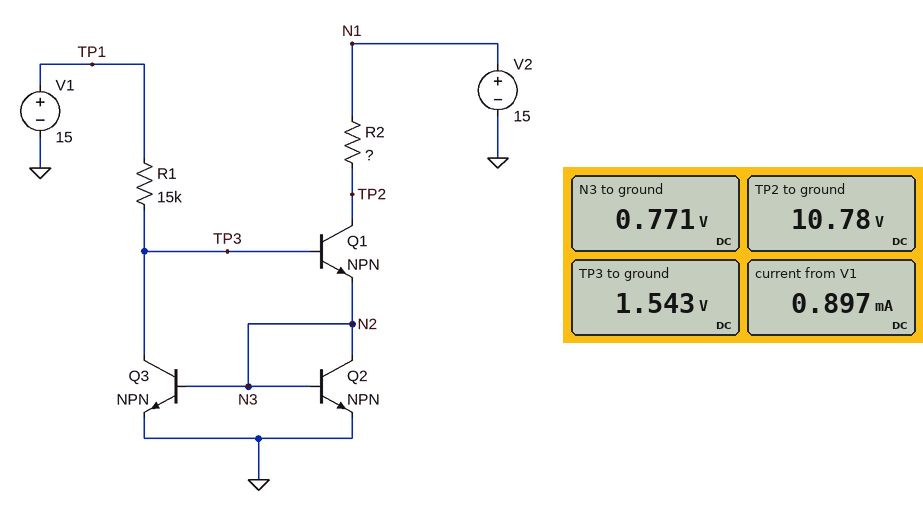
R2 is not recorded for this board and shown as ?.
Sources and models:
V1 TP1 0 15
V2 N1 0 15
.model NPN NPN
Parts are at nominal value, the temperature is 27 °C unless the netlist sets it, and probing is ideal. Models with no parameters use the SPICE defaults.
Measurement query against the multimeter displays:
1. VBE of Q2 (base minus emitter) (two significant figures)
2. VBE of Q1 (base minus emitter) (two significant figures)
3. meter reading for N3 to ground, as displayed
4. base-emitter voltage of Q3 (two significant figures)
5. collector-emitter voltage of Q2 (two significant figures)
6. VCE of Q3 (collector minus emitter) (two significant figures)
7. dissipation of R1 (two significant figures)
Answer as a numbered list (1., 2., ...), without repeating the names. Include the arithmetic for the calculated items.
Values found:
1. 771 mV = 770 mV
2. 1.543 V - 771 mV = 770 mV
3. 0.771 V
4. 771 mV = 770 mV
5. 771 mV = 770 mV
6. 1.543 V = 1.5 V
7. (15 V - 1.543 V)^2 / 15 kΩ = 12 mW
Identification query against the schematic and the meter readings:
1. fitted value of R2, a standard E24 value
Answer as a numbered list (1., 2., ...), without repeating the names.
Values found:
1. 4.7 kΩ
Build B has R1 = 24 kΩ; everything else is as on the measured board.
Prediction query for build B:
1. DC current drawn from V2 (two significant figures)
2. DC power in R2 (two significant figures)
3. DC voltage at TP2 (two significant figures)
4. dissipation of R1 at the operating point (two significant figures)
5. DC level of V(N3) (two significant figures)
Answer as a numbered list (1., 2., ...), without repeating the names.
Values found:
1. 560 µA
2. 1.5 mW
3. 12 V
4. 7.6 mW
5. 760 mV
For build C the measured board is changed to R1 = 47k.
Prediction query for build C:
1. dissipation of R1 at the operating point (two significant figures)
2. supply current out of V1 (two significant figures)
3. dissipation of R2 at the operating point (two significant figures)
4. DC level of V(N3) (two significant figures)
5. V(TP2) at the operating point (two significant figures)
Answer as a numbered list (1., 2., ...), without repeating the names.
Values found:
1. 3.9 mW
2. 290 µA
3. 390 µW
4. 740 mV
5. 14 V
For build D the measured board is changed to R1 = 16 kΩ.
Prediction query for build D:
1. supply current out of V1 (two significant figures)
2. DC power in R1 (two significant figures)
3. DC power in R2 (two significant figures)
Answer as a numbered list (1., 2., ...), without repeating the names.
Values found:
1. 840 µA
2. 11 mW
3. 3.3 mW
